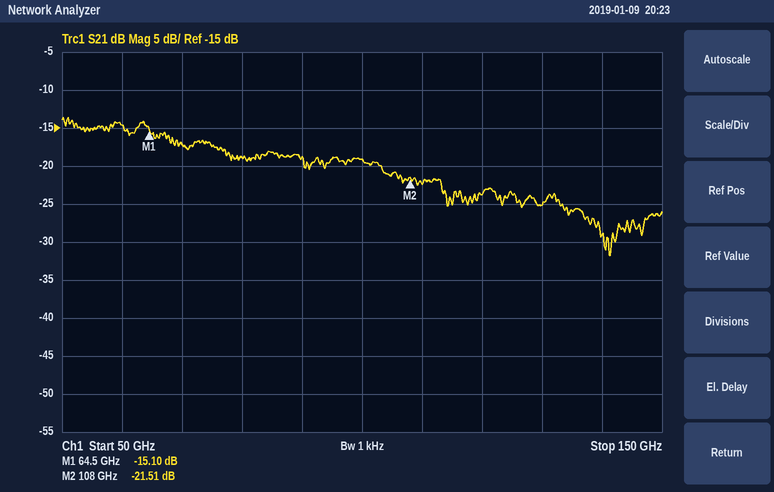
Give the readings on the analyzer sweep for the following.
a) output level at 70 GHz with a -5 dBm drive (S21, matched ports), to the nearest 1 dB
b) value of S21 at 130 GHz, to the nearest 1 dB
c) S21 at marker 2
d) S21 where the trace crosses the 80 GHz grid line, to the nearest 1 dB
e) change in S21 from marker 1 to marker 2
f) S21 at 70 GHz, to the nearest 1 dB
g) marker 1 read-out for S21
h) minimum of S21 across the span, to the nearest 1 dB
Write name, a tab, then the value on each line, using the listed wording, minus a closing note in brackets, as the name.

output level at 70 GHz with a -5 dBm drive (S21, matched ports), to the nearest 1 dB	-22 dBm
value of S21 at 130 GHz, to the nearest 1 dB	-25 dB
S21 at marker 2	-21.51 dB
S21 where the trace crosses the 80 GHz grid line, to the nearest 1 dB	-19 dB
change in S21 from marker 1 to marker 2	-6.41 dB
S21 at 70 GHz, to the nearest 1 dB	-17 dB
marker 1 read-out for S21	-15.10 dB
minimum of S21 across the span, to the nearest 1 dB	-32 dB
